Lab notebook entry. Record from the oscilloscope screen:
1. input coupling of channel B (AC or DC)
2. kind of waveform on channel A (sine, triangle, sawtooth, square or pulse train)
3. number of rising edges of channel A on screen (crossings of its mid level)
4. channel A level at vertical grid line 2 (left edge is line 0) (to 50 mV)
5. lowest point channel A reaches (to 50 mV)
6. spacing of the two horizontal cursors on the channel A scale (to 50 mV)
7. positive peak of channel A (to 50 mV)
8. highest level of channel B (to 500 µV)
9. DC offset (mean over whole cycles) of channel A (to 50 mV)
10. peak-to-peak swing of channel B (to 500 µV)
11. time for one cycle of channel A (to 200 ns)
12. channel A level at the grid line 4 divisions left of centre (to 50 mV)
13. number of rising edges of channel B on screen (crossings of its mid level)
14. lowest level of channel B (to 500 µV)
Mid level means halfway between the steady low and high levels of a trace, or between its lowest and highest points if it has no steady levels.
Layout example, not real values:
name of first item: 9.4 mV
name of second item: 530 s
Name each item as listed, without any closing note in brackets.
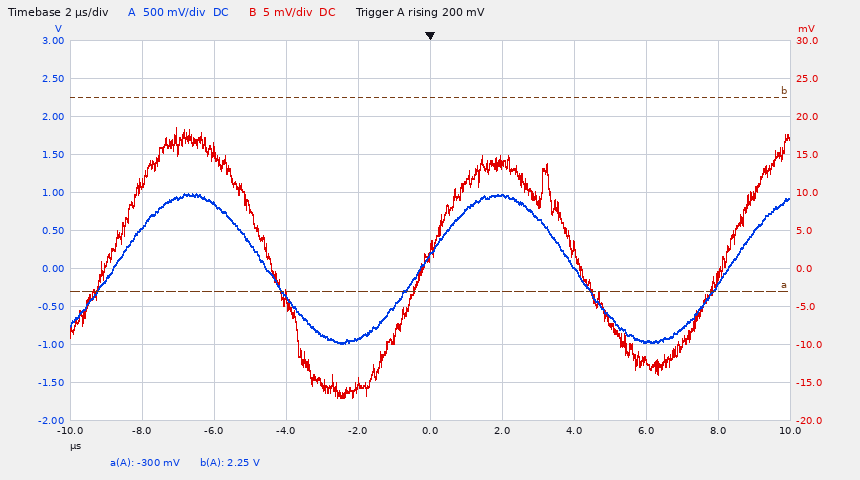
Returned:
input coupling of channel B: DC
kind of waveform on channel A: sine
number of rising edges of channel A on screen: 3
channel A level at vertical grid line 2 (left edge is line 0): 850 mV
lowest point channel A reaches: -1.00 V
spacing of the two horizontal cursors on the channel A scale: 2.55 V
positive peak of channel A: 1.00 V
highest level of channel B: 18.5 mV
DC offset (mean over whole cycles) of channel A: 0 mV
peak-to-peak swing of channel B: 35.5 mV
time for one cycle of channel A: 8.6 µs
channel A level at the grid line 4 divisions left of centre: 550 mV
number of rising edges of channel B on screen: 3
lowest level of channel B: -17.0 mV
